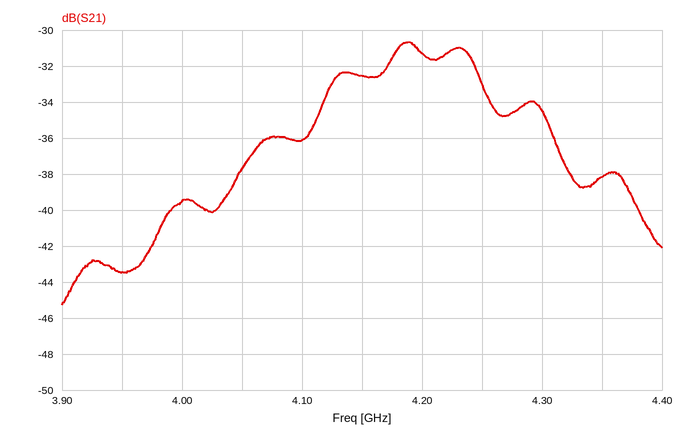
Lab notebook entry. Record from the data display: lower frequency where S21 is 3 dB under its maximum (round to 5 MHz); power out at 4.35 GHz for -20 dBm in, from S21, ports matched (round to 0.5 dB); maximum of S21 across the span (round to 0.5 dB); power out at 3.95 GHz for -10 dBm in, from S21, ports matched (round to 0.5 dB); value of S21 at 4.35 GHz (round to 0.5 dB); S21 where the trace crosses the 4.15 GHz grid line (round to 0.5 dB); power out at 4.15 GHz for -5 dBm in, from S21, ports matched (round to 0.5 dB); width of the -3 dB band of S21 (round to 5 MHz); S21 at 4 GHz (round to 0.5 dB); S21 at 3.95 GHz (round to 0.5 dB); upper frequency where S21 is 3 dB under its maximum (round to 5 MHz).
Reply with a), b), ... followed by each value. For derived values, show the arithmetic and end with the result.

a) 4.120 GHz
b) -20 dBm + (-38.0 dB) = -58.0 dBm
c) -30.5 dB
d) -10 dBm + (-43.5 dB) = -53.5 dBm
e) -38.0 dB
f) -32.5 dB
g) -5 dBm + (-32.5 dB) = -37.5 dBm
h) 4.255 GHz − 4.120 GHz = 135 MHz
i) -39.5 dB
j) -43.5 dB
k) 4.255 GHz
